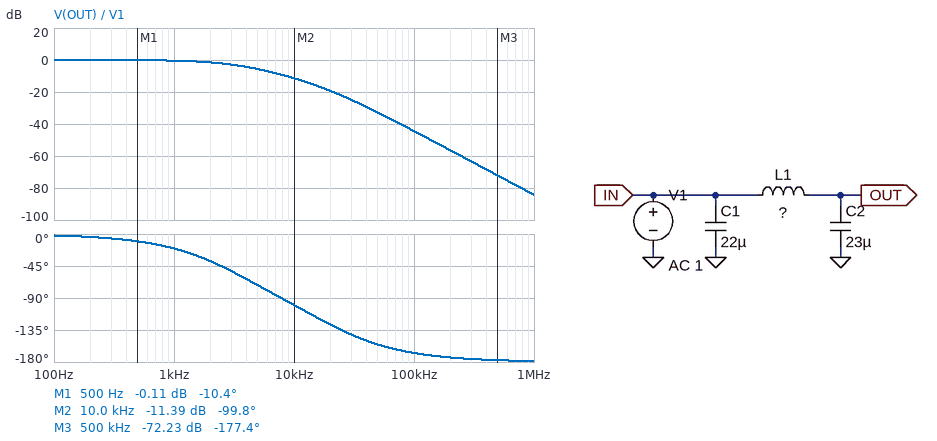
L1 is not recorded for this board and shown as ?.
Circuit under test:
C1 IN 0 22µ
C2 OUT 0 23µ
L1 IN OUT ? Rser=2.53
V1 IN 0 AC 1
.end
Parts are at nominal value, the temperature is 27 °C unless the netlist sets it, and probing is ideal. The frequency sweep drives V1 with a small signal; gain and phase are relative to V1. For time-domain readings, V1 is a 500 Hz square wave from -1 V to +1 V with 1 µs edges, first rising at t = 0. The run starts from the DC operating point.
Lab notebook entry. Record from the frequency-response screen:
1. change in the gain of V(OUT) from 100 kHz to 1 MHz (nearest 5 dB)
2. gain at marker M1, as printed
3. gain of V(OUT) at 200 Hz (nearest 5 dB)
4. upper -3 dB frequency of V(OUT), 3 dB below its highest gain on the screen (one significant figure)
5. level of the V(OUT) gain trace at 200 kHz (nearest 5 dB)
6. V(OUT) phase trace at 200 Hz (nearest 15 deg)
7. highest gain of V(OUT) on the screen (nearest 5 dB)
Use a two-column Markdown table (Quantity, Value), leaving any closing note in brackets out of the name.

| Quantity | Value |
|---|---|
| change in the gain of V(OUT) from 100 kHz to 1 MHz | -40 dB |
| gain at marker M1, as printed | -0.11 dB |
| gain of V(OUT) at 200 Hz | 0 dB |
| upper -3 dB frequency of V(OUT), 3 dB below its highest gain on the screen | 3 kHz |
| level of the V(OUT) gain trace at 200 kHz | -55 dB |
| V(OUT) phase trace at 200 Hz | 0 deg |
| highest gain of V(OUT) on the screen | 0 dB |
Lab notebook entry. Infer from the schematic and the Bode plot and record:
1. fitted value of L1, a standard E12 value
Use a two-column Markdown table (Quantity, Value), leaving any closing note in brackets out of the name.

| Quantity | Value |
|---|---|
| fitted value of L1, a standard E12 value | 18 µH |
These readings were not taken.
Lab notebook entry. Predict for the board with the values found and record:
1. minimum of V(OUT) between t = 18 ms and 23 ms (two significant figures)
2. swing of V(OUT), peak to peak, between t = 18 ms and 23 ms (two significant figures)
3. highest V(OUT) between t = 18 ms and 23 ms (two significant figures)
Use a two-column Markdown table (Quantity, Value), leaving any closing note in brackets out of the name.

| Quantity | Value |
|---|---|
| minimum of V(OUT) between t = 18 ms and 23 ms | -1.0 V |
| swing of V(OUT), peak to peak, between t = 18 ms and 23 ms | 2.0 V |
| highest V(OUT) between t = 18 ms and 23 ms | 1.0 V |
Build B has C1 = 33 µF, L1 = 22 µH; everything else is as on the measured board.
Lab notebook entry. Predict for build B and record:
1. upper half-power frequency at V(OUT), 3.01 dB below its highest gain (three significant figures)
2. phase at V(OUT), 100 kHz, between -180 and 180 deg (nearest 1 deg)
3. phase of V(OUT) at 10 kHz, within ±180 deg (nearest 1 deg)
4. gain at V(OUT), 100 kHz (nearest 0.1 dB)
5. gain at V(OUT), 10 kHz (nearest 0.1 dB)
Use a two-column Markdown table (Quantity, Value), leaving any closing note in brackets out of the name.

| Quantity | Value |
|---|---|
| upper half-power frequency at V(OUT), 3.01 dB below its highest gain | 3.20 kHz |
| phase at V(OUT), 100 kHz, between -180 and 180 deg | -170 deg |
| phase of V(OUT) at 10 kHz, within ±180 deg | -105 deg |
| gain at V(OUT), 100 kHz | -46.1 dB |
| gain at V(OUT), 10 kHz | -11.6 dB |
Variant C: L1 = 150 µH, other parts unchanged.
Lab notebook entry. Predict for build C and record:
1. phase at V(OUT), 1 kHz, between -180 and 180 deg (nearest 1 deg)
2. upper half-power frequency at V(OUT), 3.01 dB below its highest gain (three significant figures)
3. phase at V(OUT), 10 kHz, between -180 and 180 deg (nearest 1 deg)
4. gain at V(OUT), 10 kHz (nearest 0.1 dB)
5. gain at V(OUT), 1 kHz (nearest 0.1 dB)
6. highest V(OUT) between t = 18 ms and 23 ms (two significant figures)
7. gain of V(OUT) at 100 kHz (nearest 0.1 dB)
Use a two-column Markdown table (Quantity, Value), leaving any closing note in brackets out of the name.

| Quantity | Value |
|---|---|
| phase at V(OUT), 1 kHz, between -180 and 180 deg | -23 deg |
| upper half-power frequency at V(OUT), 3.01 dB below its highest gain | 3.17 kHz |
| phase at V(OUT), 10 kHz, between -180 and 180 deg | -164 deg |
| gain at V(OUT), 10 kHz | -22.4 dB |
| gain at V(OUT), 1 kHz | 0.6 dB |
| highest V(OUT) between t = 18 ms and 23 ms | 1.3 V |
| gain of V(OUT) at 100 kHz | -62.7 dB |
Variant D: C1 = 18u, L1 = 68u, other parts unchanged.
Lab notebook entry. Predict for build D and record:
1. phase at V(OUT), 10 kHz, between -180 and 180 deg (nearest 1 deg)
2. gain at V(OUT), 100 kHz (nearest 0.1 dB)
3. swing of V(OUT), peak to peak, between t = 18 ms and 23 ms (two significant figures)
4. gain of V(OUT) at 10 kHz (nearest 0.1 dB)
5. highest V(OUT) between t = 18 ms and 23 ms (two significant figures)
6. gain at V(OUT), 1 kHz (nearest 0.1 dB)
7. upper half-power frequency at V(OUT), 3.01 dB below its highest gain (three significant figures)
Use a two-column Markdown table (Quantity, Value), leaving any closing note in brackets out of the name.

| Quantity | Value |
|---|---|
| phase at V(OUT), 10 kHz, between -180 and 180 deg | -145 deg |
| gain at V(OUT), 100 kHz | -55.8 dB |
| swing of V(OUT), peak to peak, between t = 18 ms and 23 ms | 2.1 V |
| gain of V(OUT) at 10 kHz | -16.0 dB |
| highest V(OUT) between t = 18 ms and 23 ms | 1.1 V |
| gain at V(OUT), 1 kHz | -0.1 dB |
| upper half-power frequency at V(OUT), 3.01 dB below its highest gain | 3.86 kHz |
